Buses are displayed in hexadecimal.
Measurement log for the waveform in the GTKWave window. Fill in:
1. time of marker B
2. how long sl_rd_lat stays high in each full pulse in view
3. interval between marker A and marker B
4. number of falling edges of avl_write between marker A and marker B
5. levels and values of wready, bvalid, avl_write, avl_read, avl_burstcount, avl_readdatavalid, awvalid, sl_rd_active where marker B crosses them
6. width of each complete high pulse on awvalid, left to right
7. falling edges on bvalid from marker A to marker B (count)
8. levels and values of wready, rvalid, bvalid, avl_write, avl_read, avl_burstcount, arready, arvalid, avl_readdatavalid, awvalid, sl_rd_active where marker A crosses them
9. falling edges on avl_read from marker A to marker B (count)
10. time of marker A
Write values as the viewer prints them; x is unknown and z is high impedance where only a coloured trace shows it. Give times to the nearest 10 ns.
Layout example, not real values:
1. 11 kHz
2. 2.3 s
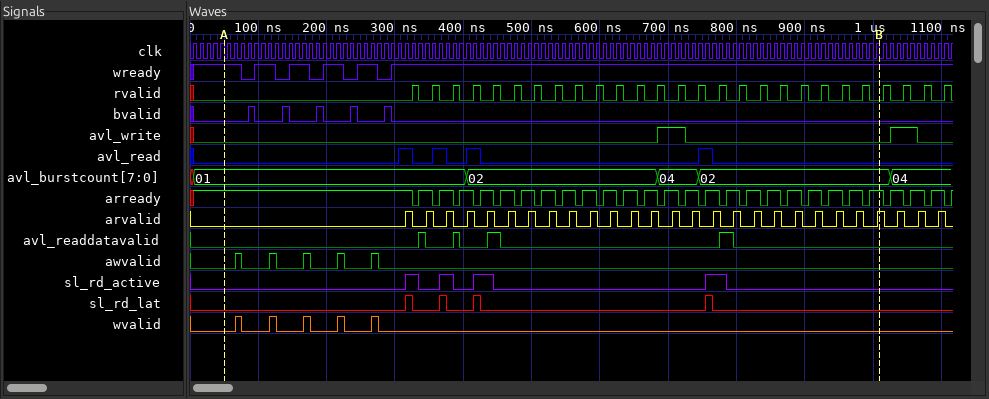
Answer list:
1. 1010 ns
2. 10 ns, 10 ns, 10 ns, 10 ns
3. 960 ns
4. 1
5. wready=1, bvalid=0, avl_write=0, avl_read=0, avl_burstcount=02, avl_readdatavalid=0, awvalid=0, sl_rd_active=0
6. 10 ns, 10 ns, 10 ns, 10 ns, 10 ns
7. 5
8. wready=1, rvalid=0, bvalid=0, avl_write=0, avl_read=0, avl_burstcount=01, arready=1, arvalid=0, avl_readdatavalid=0, awvalid=0, sl_rd_active=0
9. 4
10. 50 ns
